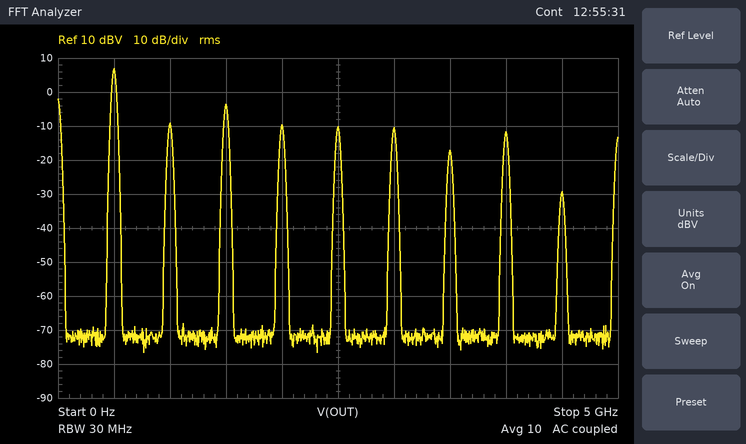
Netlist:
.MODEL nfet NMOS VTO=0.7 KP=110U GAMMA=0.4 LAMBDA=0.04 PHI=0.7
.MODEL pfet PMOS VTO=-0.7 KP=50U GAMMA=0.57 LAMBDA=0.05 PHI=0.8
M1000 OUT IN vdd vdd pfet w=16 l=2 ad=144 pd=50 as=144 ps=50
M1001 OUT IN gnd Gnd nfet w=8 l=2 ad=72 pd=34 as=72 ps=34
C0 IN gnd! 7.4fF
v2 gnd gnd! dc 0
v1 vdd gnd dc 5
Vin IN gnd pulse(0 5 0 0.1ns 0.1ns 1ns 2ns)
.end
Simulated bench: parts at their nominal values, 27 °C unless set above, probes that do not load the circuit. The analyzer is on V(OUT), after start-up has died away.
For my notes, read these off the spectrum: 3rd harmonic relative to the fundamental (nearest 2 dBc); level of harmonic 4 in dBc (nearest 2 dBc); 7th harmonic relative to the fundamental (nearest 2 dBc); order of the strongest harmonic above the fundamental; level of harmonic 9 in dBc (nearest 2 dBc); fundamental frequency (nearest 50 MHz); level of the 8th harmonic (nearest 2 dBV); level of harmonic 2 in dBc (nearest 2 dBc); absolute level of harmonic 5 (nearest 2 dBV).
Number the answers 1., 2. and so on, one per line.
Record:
1. -10 dBc
2. -16 dBc
3. -24 dBc
4. 3
5. -36 dBc
6. 500 MHz
7. -12 dBV
8. -16 dBc
9. -10 dBV
